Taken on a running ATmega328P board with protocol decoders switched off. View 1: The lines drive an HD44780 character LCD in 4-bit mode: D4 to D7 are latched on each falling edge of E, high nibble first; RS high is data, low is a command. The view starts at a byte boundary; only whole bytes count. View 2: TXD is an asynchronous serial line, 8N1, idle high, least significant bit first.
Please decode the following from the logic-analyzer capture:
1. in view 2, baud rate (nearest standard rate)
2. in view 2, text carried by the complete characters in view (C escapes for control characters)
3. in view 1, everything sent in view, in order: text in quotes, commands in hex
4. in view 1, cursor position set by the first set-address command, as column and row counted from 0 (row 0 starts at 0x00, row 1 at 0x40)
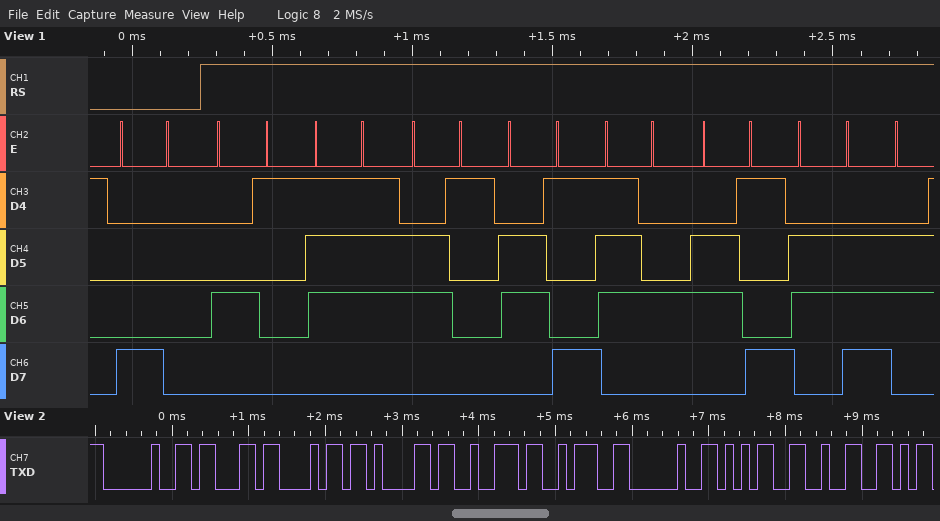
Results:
9600 baud
" char: 52"
0x80 "Awaitin"
column 0, row 0
